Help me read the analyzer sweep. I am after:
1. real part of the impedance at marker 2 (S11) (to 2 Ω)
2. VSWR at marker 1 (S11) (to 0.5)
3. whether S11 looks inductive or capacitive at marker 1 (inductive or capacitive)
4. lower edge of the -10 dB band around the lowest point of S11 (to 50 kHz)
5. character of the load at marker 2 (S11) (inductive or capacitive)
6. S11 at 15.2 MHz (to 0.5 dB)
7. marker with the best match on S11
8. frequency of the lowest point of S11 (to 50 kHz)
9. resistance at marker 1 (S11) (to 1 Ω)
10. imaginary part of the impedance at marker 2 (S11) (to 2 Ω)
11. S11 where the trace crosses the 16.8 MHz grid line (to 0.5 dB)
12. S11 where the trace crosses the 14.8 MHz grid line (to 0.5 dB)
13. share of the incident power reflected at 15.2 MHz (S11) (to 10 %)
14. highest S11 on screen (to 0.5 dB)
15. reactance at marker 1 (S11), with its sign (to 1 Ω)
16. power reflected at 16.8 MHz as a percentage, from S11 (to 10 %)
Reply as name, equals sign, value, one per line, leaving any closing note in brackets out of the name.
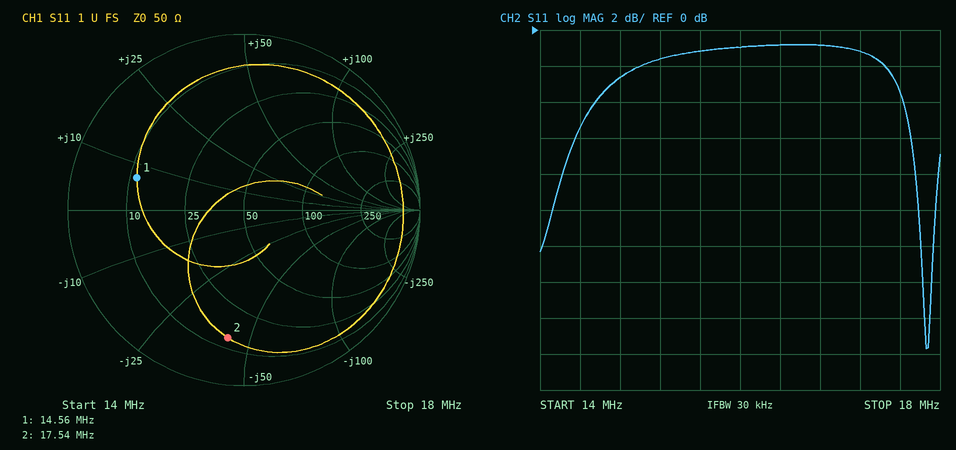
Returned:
real part of the impedance at marker 2 (S11) = 14 Ω
VSWR at marker 1 (S11) = 4.5
whether S11 looks inductive or capacitive at marker 1 = inductive
lower edge of the -10 dB band around the lowest point of S11 = 17.80 MHz
character of the load at marker 2 (S11) = capacitive
S11 at 15.2 MHz = -1.5 dB
marker with the best match on S11 = marker 1
frequency of the lowest point of S11 = 17.85 MHz
resistance at marker 1 (S11) = 11 Ω
imaginary part of the impedance at marker 2 (S11) = -42 Ω
S11 where the trace crosses the 16.8 MHz grid line = -1.0 dB
S11 where the trace crosses the 14.8 MHz grid line = -2.5 dB
share of the incident power reflected at 15.2 MHz (S11) = 70 %
highest S11 on screen = -1.0 dB
reactance at marker 1 (S11), with its sign = +7 Ω
power reflected at 16.8 MHz as a percentage, from S11 = 80 %
